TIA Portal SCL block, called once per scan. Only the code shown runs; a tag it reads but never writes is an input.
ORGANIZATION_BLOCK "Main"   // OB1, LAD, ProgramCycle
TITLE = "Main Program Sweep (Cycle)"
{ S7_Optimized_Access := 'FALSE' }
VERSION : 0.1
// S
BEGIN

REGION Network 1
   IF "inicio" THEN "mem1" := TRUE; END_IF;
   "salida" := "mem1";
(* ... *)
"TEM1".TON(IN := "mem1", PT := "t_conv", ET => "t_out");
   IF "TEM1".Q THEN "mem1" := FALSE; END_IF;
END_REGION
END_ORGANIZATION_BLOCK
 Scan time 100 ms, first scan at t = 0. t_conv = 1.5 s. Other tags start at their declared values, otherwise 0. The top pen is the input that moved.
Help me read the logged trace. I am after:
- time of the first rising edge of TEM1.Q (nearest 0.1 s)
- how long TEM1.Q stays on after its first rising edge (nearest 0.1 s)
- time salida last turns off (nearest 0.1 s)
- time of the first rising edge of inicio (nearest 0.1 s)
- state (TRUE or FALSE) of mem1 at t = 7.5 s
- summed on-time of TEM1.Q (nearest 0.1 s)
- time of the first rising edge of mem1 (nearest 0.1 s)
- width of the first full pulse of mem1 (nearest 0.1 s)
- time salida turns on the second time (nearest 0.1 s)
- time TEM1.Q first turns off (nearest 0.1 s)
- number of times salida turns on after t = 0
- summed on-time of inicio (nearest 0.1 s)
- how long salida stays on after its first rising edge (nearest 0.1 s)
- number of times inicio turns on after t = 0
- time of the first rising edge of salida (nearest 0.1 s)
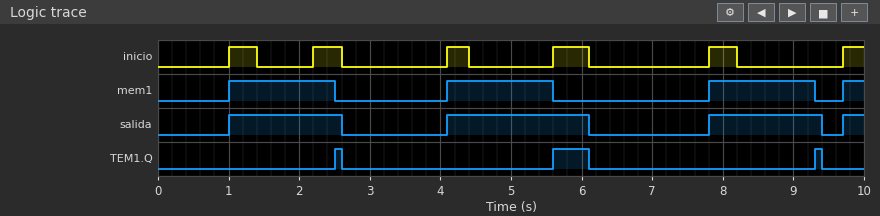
2.5 s
0.1 s
9.4 s
1.0 s
FALSE
0.7 s
1.0 s
1.5 s
4.1 s
2.6 s
4
2.3 s
1.6 s
6
1.0 s
